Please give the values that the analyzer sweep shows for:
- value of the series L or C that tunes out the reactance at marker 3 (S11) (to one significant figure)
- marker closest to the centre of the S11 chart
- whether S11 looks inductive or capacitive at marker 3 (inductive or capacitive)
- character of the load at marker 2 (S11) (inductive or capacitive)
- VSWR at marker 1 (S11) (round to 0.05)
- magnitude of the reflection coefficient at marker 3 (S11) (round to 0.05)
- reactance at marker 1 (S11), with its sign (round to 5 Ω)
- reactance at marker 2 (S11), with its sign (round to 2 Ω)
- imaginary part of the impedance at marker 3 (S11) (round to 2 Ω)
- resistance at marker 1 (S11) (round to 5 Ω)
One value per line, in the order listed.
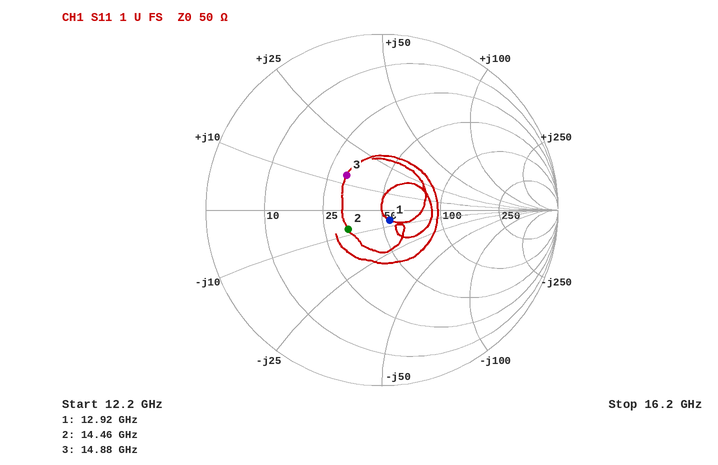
800 fF
marker 1
inductive
capacitive
1.15
0.30
-5 Ω
-8 Ω
+14 Ω
55 Ω
